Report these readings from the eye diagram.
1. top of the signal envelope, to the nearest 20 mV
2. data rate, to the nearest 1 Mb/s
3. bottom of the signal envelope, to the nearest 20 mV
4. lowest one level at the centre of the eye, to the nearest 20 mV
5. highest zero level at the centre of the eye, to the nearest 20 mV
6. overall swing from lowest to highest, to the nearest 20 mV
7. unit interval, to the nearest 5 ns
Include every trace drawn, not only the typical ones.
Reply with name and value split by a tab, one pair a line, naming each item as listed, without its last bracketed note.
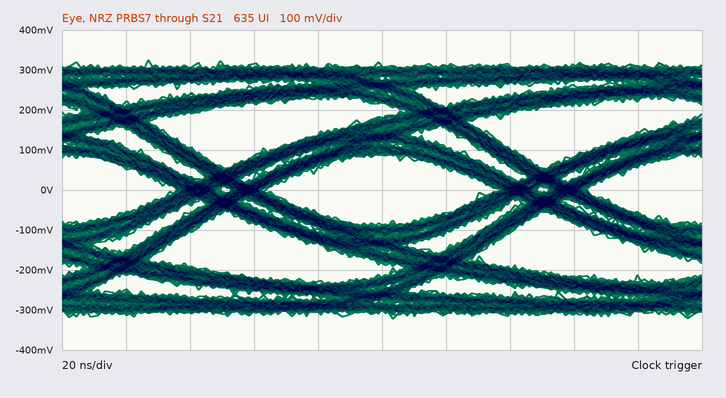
top of the signal envelope, to the nearest 20 mV	320 mV
data rate, to the nearest 1 Mb/s	10 Mb/s
bottom of the signal envelope, to the nearest 20 mV	-320 mV
lowest one level at the centre of the eye, to the nearest 20 mV	80 mV
highest zero level at the centre of the eye, to the nearest 20 mV	-80 mV
overall swing from lowest to highest, to the nearest 20 mV	640 mV
unit interval, to the nearest 5 ns	100 ns
